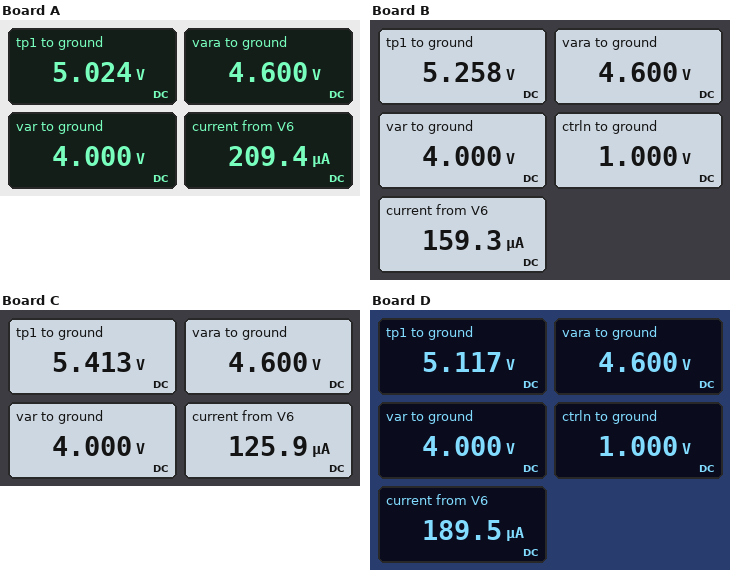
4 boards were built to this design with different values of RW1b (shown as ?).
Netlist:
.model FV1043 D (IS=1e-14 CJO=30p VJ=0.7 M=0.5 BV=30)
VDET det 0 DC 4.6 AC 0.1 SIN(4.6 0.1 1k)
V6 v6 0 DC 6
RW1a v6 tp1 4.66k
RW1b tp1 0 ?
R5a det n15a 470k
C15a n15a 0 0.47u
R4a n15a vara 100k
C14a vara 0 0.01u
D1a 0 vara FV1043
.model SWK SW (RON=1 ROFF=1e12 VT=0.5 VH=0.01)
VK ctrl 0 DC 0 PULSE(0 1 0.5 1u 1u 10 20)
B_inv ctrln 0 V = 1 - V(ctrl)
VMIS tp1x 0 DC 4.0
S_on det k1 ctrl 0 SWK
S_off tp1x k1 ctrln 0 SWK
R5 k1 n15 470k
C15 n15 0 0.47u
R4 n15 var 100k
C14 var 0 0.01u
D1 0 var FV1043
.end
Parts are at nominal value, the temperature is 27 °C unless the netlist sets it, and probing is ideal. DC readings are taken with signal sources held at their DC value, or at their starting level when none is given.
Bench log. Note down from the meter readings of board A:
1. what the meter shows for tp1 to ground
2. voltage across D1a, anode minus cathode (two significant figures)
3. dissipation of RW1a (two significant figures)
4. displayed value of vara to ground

5.024 V
-4.6 V
200 µW
4.600 V
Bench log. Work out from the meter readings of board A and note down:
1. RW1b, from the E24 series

24 kΩ
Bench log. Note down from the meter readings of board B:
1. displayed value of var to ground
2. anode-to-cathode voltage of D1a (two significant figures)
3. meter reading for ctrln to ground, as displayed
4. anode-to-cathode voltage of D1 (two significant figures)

4.000 V
-4.6 V
1.000 V
-4.0 V
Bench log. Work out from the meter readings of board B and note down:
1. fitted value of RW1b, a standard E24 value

33 kΩ
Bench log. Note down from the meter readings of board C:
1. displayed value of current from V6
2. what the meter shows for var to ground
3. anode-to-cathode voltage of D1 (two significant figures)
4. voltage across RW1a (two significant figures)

125.9 µA
4.000 V
-4.0 V
590 mV
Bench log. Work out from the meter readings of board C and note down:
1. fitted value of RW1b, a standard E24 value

43 kΩ
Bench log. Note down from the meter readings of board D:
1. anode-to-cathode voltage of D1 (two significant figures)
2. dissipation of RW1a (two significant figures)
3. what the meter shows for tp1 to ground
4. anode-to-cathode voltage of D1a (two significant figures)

-4.0 V
170 µW
5.117 V
-4.6 V
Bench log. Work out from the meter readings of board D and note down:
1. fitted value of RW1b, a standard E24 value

27 kΩ
